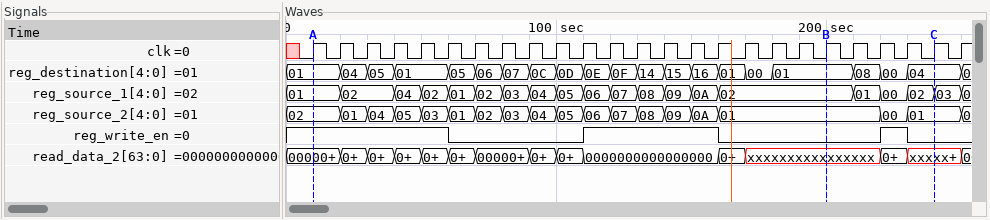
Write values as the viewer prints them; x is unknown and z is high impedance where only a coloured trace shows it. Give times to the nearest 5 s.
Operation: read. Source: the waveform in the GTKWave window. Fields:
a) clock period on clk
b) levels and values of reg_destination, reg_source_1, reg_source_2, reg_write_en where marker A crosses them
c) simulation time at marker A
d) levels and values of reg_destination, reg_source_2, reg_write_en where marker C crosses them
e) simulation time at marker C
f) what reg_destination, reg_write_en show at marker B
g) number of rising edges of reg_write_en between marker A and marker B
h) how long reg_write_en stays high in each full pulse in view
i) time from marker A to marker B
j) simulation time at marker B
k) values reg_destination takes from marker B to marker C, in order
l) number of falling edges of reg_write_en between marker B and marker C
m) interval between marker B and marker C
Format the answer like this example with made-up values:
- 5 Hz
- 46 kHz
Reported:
- 10 s
- reg_destination=01, reg_source_1=01, reg_source_2=02, reg_write_en=1
- 10 s
- reg_destination=04, reg_source_2=01, reg_write_en=0
- 240 s
- reg_destination=01, reg_write_en=0
- 1
- 50 s, 10 s
- 190 s
- 200 s
- 01, 08, 00, 04
- 1
- 40 s
